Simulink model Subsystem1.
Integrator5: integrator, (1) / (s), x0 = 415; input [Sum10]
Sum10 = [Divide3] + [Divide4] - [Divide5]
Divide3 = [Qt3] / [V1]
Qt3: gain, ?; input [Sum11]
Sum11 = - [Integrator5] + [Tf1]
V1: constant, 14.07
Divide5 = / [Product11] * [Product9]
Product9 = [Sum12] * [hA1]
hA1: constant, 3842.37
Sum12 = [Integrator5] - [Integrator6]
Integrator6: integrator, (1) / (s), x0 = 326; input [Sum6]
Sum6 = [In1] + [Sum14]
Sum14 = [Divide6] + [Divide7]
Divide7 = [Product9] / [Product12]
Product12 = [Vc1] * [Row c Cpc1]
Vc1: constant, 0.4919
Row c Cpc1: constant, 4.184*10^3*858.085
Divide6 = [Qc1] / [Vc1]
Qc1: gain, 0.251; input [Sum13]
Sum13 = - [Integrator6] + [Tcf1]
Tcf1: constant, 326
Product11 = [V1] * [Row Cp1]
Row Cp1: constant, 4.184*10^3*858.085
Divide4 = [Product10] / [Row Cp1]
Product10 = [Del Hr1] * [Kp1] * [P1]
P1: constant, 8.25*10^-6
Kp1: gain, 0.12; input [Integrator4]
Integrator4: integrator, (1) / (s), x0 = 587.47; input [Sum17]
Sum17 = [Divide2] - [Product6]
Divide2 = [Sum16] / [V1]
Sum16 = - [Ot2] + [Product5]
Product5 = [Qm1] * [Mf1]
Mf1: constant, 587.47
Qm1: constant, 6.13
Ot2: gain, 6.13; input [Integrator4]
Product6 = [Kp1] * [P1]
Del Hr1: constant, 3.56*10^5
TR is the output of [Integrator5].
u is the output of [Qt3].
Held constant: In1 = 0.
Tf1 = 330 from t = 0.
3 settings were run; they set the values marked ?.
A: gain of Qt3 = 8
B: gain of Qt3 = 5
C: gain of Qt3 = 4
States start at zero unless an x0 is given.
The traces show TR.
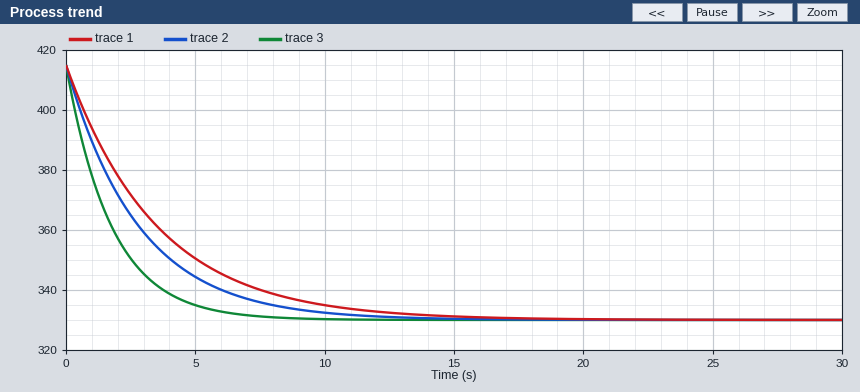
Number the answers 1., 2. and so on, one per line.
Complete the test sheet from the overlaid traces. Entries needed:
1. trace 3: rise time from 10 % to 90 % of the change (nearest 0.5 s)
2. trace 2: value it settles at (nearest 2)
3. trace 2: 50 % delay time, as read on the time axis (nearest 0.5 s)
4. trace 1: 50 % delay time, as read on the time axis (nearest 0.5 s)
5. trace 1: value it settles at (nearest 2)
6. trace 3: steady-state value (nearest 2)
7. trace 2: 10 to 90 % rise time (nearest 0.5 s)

1. 4.0 s
2. 330
3. 2.0 s
4. 2.5 s
5. 330
6. 330
7. 6.0 s
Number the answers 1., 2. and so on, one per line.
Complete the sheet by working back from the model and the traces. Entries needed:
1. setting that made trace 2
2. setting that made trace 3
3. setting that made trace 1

1. B
2. A
3. C
